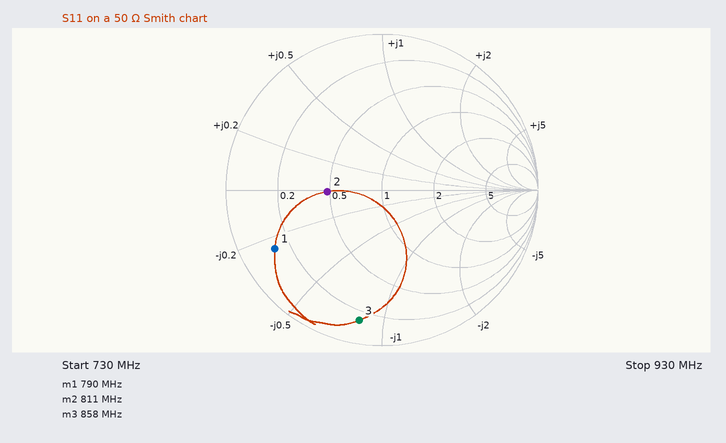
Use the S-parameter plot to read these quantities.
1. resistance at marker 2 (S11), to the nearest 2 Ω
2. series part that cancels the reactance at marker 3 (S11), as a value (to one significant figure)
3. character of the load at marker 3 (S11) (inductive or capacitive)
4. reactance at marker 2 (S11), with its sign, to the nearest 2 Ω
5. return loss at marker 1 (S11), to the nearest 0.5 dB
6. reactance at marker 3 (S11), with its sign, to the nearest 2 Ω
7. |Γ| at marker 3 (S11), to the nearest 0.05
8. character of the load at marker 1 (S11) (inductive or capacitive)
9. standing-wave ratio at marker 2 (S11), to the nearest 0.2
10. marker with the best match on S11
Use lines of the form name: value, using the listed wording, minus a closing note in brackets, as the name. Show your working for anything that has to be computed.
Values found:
resistance at marker 2 (S11), to the nearest 2 Ω: 24 Ω
series part that cancels the reactance at marker 3 (S11), as a value: L = 42 Ω/(2π × 858 MHz) ≈ 8 nH
character of the load at marker 3 (S11): capacitive
reactance at marker 2 (S11), with its sign, to the nearest 2 Ω: 0 Ω
return loss at marker 1 (S11), to the nearest 0.5 dB: 2.0 dB
reactance at marker 3 (S11), with its sign, to the nearest 2 Ω: -42 Ω
|Γ| at marker 3 (S11), to the nearest 0.05: 0.85
character of the load at marker 1 (S11): capacitive
standing-wave ratio at marker 2 (S11), to the nearest 0.2: 2.0
marker with the best match on S11: marker 2
